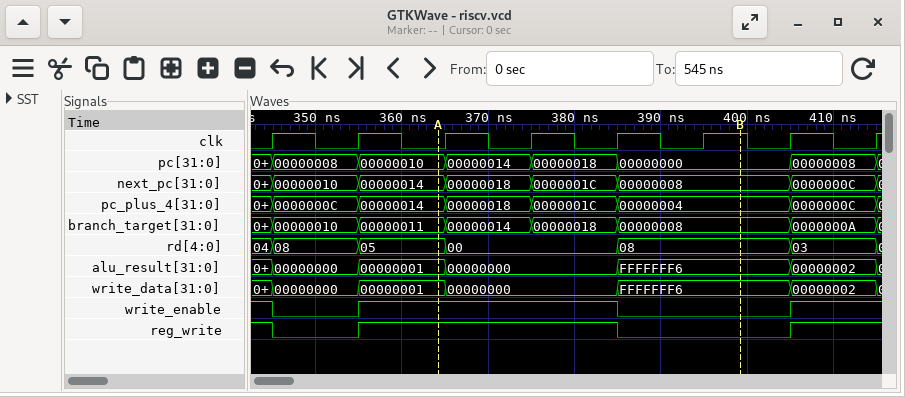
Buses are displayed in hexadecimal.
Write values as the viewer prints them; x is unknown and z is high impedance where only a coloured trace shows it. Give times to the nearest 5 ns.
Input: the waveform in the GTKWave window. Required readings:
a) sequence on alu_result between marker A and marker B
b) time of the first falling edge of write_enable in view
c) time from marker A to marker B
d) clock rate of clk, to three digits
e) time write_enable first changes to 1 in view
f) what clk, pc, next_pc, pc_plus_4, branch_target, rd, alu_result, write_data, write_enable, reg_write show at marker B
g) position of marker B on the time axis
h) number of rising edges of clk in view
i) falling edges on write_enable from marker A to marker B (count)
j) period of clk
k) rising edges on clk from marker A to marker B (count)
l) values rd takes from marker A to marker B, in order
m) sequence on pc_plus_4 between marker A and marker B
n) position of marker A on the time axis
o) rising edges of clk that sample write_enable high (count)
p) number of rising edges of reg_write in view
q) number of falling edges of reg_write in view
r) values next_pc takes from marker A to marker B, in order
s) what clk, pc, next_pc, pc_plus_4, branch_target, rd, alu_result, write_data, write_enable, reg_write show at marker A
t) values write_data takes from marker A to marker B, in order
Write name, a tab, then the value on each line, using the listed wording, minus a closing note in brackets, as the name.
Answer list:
sequence on alu_result between marker A and marker B	00000001, 00000000, FFFFFFF6
time of the first falling edge of write_enable in view	345 ns
time from marker A to marker B	35 ns
clock rate of clk, to three digits	100 MHz
time write_enable first changes to 1 in view	355 ns
what clk, pc, next_pc, pc_plus_4, branch_target, rd, alu_result, write_data, write_enable, reg_write show at marker B	clk=1, pc=00000000, next_pc=00000008, pc_plus_4=00000004, branch_target=00000008, rd=08, alu_result=FFFFFFF6, write_data=FFFFFFF6, write_enable=0, reg_write=0
position of marker B on the time axis	400 ns
number of rising edges of clk in view	8
falling edges on write_enable from marker A to marker B	1
period of clk	10 ns
rising edges on clk from marker A to marker B	4
values rd takes from marker A to marker B, in order	05, 00, 08
sequence on pc_plus_4 between marker A and marker B	00000014, 00000018, 0000001C, 00000004
position of marker A on the time axis	365 ns
rising edges of clk that sample write_enable high	5
number of rising edges of reg_write in view	2
number of falling edges of reg_write in view	2
values next_pc takes from marker A to marker B, in order	00000014, 00000018, 0000001C, 00000008
what clk, pc, next_pc, pc_plus_4, branch_target, rd, alu_result, write_data, write_enable, reg_write show at marker A	clk=0, pc=00000010, next_pc=00000014, pc_plus_4=00000014, branch_target=00000011, rd=05, alu_result=00000001, write_data=00000001, write_enable=1, reg_write=1
values write_data takes from marker A to marker B, in order	00000001, 00000000, FFFFFFF6
